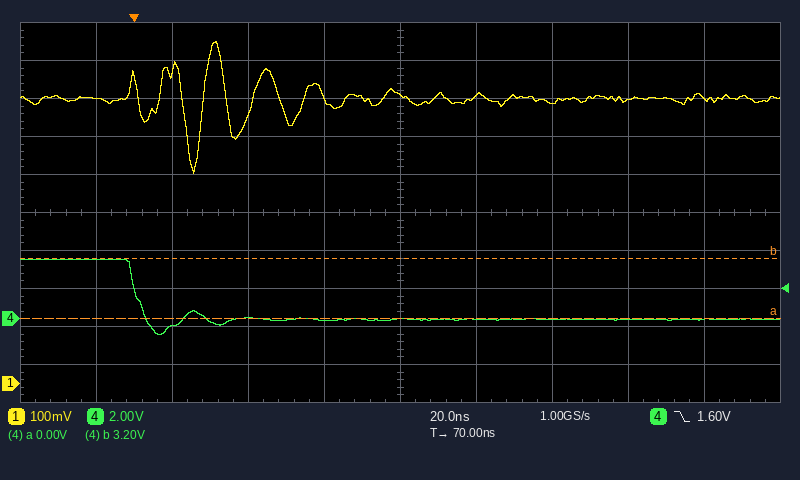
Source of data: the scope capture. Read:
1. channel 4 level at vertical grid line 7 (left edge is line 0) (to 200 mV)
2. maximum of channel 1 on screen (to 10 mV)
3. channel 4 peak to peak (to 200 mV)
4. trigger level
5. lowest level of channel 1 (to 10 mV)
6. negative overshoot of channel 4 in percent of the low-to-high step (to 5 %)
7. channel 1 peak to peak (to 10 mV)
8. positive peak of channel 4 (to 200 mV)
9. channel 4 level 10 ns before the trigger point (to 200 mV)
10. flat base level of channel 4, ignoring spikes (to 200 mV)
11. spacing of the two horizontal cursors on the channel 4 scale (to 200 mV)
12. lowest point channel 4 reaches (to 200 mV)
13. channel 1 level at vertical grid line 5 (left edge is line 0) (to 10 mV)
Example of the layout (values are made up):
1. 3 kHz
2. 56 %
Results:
1. 0.0 V
2. 900 mV
3. 4.0 V
4. 1.60 V
5. 550 mV
6. 25 %
7. 350 mV
8. 3.2 V
9. 3.2 V
10. 0.0 V
11. 3.2 V
12. -800 mV
13. 760 mV
